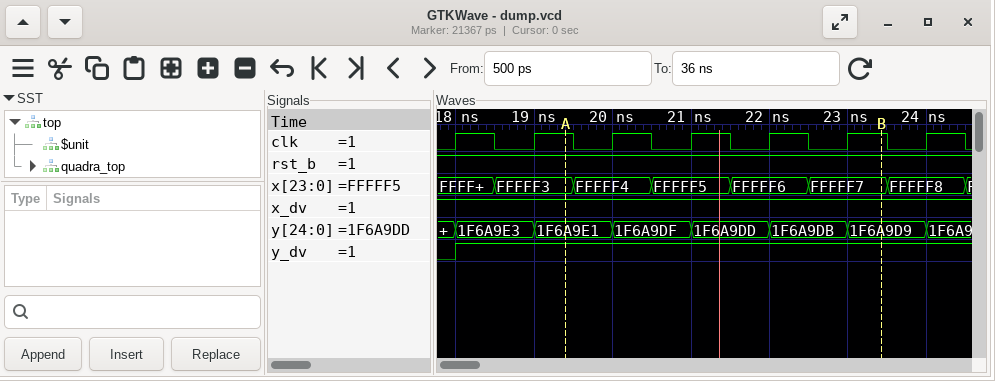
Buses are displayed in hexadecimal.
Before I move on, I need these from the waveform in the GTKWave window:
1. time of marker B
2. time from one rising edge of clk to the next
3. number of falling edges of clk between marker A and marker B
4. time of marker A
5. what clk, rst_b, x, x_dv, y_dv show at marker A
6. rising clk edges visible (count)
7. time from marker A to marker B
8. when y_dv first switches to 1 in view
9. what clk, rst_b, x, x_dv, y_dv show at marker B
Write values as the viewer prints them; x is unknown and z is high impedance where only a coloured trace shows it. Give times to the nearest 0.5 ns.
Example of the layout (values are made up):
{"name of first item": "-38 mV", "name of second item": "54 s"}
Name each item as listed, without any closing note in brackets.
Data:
{"time of marker B": "23.5 ns", "time from one rising edge of clk to the next": "1 ns", "number of falling edges of clk between marker A and marker B": "4", "time of marker A": "19.5 ns", "what clk, rst_b, x, x_dv, y_dv show at marker A": "clk=1, rst_b=1, x=FFFFF3, x_dv=1, y_dv=1", "rising clk edges visible": "7", "time from marker A to marker B": "4 ns", "when y_dv first switches to 1 in view": "18 ns", "what clk, rst_b, x, x_dv, y_dv show at marker B": "clk=1, rst_b=1, x=FFFFF7, x_dv=1, y_dv=1"}
